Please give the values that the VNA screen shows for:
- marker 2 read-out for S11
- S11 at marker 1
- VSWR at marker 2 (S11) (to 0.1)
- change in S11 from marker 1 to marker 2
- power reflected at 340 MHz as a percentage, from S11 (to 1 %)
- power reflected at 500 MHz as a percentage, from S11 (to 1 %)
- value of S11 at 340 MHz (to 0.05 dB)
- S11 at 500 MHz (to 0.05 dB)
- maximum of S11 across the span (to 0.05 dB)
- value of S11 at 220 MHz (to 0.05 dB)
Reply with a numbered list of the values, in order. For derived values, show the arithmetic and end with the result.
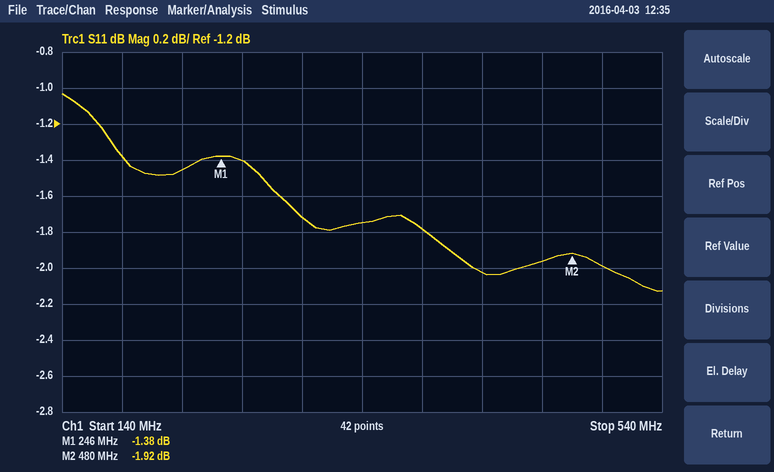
1. -1.92 dB
2. -1.38 dB
3. (1 + 0.8017)/(1 − 0.8017) ≈ 9.1
4. -1.92 − (-1.38) = -0.54 dB
5. 10^(-1.75/10) ≈ 67 %
6. 10^(-2/10) ≈ 63 %
7. -1.75 dB
8. -2.00 dB
9. -1.05 dB
10. -1.45 dB
